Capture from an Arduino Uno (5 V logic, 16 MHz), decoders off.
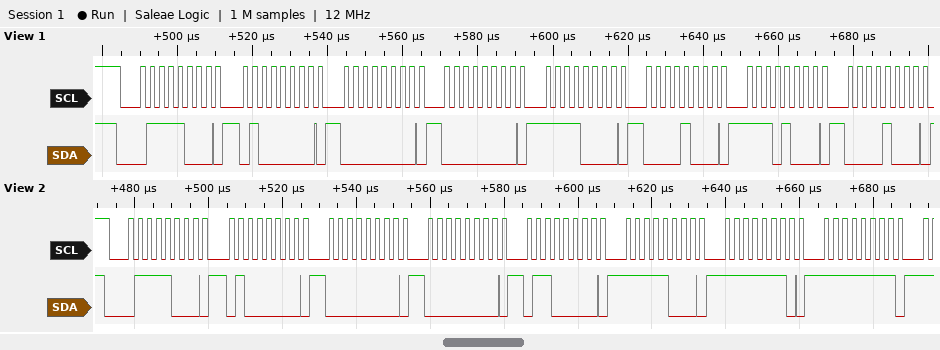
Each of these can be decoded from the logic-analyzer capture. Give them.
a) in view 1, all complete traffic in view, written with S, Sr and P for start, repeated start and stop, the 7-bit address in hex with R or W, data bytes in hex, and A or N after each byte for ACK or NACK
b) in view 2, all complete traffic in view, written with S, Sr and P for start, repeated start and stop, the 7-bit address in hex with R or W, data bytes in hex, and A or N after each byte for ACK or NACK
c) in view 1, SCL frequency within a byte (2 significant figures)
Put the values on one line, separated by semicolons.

S 3CW A 40 A 00 A 00 A F0 A 08 A E8 A 08 A; S 3CW A 40 A 00 A 00 A 60 A F8 A FE A FF A; 400 kHz
